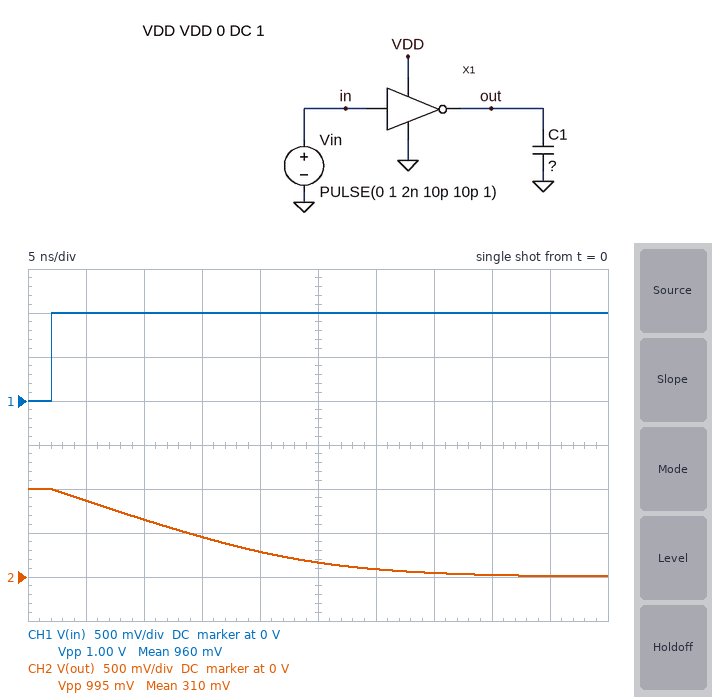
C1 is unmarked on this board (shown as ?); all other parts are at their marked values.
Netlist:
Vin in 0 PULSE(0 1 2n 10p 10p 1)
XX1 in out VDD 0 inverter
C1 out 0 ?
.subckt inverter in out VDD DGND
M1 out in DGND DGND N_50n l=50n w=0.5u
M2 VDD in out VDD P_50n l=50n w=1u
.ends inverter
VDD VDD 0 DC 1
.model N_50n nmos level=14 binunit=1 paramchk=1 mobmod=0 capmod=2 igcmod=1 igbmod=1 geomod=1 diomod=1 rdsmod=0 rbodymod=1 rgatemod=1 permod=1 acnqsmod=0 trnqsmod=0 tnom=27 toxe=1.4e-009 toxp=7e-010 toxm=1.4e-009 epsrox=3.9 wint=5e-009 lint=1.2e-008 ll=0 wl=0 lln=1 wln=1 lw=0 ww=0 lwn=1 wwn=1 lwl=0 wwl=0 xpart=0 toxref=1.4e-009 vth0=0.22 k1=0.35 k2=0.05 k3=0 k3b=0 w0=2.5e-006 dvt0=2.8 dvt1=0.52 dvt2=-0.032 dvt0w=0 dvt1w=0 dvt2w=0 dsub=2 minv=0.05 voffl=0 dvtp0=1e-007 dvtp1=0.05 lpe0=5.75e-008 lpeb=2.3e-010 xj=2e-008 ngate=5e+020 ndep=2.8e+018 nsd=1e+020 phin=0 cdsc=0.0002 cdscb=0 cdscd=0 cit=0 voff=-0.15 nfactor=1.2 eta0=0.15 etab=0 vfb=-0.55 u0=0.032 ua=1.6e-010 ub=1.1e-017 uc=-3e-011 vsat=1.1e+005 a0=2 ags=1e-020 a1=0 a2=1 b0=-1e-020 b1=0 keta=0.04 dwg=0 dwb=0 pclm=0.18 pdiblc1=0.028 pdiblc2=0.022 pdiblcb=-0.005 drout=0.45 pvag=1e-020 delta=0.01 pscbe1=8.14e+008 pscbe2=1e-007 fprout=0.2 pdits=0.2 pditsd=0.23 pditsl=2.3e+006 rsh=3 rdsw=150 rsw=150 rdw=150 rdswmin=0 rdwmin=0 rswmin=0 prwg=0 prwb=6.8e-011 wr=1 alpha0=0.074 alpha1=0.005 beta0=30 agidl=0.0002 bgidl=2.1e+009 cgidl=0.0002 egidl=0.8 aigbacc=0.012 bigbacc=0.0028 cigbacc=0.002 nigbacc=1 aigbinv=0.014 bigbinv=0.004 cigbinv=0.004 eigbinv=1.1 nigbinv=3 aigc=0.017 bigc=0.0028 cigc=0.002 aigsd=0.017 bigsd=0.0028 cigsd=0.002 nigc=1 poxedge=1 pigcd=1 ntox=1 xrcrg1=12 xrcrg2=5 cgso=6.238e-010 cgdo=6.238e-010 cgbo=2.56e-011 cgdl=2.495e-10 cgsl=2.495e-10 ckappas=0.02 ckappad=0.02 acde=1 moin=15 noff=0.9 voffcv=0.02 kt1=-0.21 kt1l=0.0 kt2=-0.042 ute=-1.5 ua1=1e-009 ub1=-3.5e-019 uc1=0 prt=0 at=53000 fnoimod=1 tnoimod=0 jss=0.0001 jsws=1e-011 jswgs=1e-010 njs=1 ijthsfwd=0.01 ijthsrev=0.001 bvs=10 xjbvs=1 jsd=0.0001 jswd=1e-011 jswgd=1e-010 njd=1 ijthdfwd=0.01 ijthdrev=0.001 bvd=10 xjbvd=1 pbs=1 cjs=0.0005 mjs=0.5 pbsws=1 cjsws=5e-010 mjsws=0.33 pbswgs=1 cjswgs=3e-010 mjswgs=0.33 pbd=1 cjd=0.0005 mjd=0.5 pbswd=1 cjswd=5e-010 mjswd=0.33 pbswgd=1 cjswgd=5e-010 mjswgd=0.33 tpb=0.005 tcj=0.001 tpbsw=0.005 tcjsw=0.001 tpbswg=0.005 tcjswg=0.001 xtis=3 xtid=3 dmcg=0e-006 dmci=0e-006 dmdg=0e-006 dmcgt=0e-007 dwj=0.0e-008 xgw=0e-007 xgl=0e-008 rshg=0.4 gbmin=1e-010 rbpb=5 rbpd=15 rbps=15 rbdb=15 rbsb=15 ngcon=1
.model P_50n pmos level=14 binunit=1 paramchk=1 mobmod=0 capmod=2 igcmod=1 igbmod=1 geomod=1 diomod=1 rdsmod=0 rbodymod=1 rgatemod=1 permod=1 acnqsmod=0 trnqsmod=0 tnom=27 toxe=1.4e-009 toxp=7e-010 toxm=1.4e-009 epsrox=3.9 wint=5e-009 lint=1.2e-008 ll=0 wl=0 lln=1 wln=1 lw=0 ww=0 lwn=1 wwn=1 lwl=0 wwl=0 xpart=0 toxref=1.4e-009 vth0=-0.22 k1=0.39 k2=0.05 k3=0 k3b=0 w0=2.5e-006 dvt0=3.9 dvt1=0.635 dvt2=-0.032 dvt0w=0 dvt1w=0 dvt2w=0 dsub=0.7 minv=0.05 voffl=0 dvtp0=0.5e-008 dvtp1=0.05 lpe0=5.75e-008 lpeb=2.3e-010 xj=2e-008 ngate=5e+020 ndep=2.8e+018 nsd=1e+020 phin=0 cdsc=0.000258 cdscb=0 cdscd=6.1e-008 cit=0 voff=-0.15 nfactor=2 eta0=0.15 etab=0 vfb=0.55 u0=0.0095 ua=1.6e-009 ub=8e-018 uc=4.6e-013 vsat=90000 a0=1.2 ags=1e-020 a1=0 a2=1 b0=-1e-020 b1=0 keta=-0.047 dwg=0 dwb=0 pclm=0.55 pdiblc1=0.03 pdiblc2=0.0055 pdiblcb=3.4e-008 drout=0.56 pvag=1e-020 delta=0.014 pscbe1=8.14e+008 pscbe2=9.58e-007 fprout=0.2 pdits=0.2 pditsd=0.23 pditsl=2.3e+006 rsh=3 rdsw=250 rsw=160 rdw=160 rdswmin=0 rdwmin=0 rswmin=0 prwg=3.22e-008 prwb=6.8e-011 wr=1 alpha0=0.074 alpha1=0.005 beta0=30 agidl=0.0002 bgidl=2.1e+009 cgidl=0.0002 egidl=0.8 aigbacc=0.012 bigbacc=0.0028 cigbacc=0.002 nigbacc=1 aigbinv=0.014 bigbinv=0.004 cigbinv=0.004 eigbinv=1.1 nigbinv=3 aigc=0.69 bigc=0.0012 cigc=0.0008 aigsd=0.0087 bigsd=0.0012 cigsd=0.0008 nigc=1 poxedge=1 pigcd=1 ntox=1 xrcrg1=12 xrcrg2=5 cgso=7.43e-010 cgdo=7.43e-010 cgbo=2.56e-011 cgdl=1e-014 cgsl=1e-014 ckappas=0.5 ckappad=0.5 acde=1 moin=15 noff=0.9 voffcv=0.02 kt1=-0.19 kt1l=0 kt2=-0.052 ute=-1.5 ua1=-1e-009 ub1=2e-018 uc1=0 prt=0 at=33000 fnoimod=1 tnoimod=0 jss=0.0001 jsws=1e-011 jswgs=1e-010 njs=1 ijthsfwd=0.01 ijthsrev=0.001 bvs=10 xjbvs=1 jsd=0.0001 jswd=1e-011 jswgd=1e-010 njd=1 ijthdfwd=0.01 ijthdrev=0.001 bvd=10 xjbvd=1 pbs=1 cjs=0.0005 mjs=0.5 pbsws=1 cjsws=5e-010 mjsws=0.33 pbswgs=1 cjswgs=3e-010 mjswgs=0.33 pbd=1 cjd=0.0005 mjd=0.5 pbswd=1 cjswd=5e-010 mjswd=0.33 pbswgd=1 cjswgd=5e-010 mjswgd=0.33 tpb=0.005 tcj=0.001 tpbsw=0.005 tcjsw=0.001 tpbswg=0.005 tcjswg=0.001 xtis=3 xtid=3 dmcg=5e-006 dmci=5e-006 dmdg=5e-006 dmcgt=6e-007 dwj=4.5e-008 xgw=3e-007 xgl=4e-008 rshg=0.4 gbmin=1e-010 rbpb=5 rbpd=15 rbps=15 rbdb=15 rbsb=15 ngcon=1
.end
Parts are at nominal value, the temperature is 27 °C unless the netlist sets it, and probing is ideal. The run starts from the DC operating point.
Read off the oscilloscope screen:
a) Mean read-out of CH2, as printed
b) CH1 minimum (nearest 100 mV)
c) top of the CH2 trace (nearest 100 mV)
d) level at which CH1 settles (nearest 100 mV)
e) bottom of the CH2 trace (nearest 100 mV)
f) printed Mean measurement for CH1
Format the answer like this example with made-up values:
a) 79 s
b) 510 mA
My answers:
a) 310 mV
b) 0 V
c) 1.0 V
d) 1.0 V
e) 0 V
f) 960 mV
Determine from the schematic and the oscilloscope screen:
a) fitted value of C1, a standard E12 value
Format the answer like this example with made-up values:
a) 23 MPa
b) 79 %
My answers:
a) 6.8 pF
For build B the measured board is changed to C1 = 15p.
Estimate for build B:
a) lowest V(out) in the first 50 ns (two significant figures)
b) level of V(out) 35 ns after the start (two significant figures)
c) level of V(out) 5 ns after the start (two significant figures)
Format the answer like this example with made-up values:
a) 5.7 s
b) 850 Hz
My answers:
a) 190 mV
b) 380 mV
c) 940 mV
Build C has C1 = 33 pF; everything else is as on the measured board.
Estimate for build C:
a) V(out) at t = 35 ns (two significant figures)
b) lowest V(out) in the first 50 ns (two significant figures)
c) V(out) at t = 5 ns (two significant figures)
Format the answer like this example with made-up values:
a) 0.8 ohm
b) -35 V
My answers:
a) 700 mV
b) 570 mV
c) 970 mV
